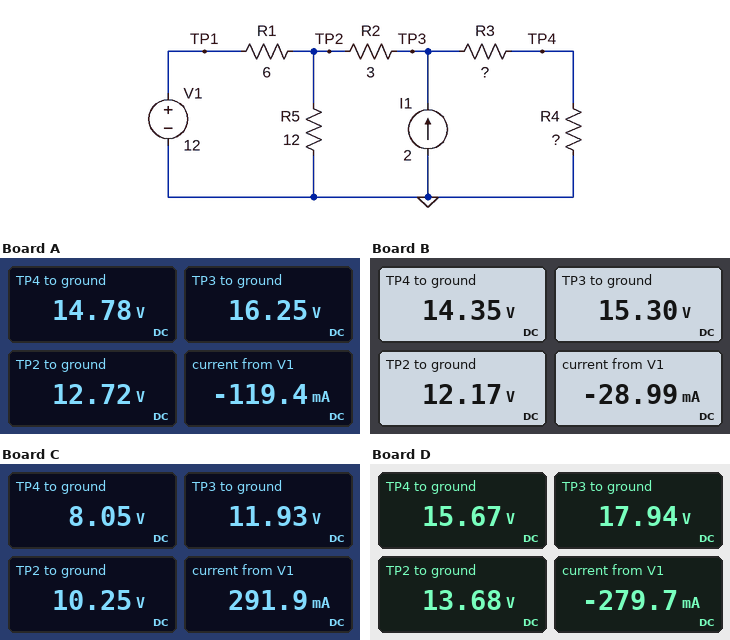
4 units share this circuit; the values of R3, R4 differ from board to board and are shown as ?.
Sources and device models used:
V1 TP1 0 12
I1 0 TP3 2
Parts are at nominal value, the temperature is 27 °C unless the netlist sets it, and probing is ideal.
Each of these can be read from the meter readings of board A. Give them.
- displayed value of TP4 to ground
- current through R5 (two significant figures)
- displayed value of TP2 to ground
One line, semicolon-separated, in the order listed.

14.78 V; 1.1 A; 12.72 V
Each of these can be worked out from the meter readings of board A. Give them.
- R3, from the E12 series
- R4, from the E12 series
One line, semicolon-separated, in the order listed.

1.8 Ω; 18 Ω
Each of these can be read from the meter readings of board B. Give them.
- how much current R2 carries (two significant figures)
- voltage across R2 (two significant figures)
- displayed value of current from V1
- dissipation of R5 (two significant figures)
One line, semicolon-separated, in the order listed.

1.0 A; 3.1 V; -28.99 mA; 12 W
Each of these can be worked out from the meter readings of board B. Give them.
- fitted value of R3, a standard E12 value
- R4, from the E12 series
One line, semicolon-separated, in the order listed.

1 Ω; 15 Ω
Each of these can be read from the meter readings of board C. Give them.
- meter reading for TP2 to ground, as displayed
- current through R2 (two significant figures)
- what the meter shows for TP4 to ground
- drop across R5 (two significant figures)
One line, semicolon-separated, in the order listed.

10.25 V; 560 mA; 8.05 V; 10 V
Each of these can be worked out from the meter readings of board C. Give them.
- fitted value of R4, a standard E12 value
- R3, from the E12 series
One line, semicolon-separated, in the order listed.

5.6 Ω; 2.7 Ω
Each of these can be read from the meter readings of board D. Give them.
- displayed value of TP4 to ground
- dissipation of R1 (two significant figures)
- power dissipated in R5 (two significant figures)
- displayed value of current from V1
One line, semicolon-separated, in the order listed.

15.67 V; 470 mW; 16 W; -279.7 mA
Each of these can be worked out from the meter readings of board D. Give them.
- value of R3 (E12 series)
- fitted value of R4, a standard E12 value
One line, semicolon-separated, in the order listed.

3.9 Ω; 27 Ω
